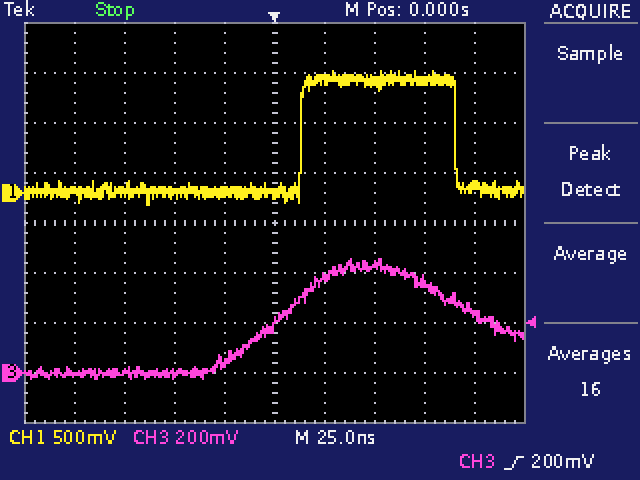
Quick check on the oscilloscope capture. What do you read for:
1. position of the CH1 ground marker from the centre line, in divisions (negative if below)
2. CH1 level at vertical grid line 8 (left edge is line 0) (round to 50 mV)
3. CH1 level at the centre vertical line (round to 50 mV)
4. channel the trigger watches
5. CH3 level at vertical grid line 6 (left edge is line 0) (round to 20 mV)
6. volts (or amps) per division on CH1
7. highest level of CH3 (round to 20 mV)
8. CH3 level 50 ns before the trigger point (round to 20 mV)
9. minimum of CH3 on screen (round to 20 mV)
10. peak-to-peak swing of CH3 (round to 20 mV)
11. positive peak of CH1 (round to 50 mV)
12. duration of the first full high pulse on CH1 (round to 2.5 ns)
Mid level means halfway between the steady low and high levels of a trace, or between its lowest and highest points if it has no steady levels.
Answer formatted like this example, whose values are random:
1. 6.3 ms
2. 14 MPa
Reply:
1. +0.6 div
2. 1.10 V
3. 0 mV
4. CH3
5. 380 mV
6. 500 mV
7. 460 mV
8. 0 mV
9. -20 mV
10. 480 mV
11. 1.20 V
12. 77.5 ns
